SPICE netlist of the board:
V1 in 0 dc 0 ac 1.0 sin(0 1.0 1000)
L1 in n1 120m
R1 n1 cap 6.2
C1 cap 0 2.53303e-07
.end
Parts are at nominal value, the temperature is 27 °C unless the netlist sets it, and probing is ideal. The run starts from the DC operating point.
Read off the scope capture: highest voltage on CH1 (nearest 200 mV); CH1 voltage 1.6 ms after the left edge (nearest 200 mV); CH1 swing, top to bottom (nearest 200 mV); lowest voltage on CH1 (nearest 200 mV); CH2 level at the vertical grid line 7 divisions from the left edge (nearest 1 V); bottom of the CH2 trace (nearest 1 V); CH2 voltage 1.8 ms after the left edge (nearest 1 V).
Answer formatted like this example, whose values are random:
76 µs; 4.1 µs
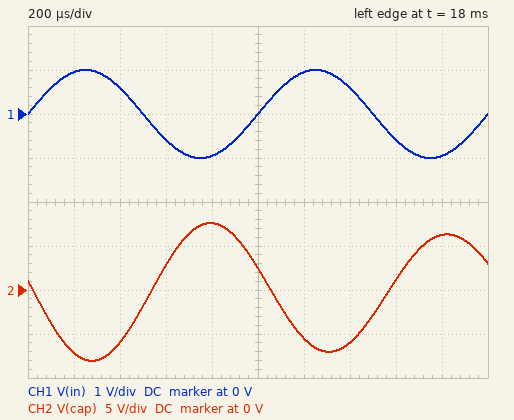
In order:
1.0 V; -600 mV; 2.0 V; -1.0 V; -6 V; -8 V; 6 V
